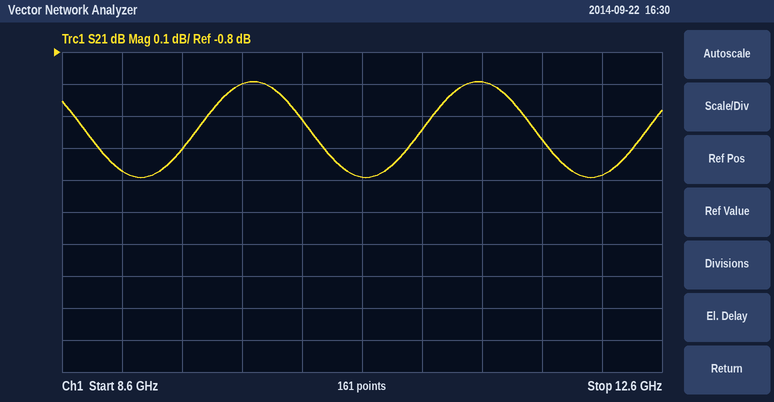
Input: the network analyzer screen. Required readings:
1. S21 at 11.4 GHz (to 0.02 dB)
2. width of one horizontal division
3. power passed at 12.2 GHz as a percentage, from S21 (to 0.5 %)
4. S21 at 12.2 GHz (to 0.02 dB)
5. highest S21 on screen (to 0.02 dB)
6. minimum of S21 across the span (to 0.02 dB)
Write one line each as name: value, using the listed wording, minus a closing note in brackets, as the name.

S21 at 11.4 GHz: -0.90 dB
width of one horizontal division: 400 MHz
power passed at 12.2 GHz as a percentage, from S21: 76.0 %
S21 at 12.2 GHz: -1.18 dB
highest S21 on screen: -0.90 dB
minimum of S21 across the span: -1.20 dB
